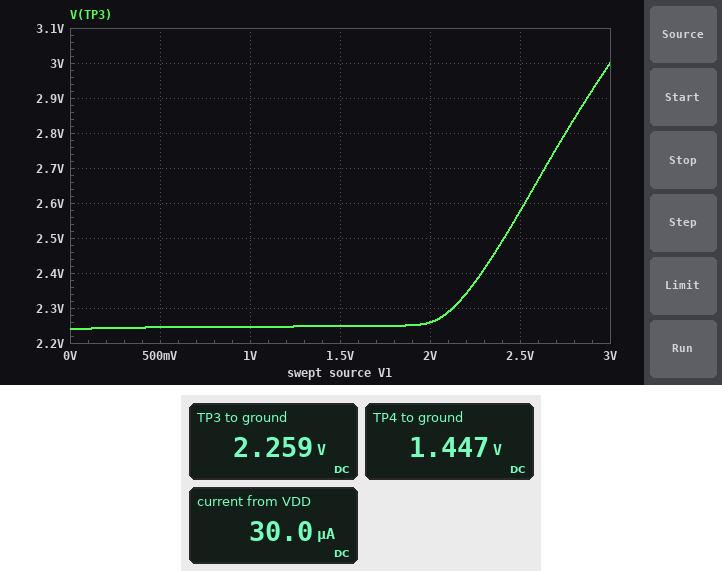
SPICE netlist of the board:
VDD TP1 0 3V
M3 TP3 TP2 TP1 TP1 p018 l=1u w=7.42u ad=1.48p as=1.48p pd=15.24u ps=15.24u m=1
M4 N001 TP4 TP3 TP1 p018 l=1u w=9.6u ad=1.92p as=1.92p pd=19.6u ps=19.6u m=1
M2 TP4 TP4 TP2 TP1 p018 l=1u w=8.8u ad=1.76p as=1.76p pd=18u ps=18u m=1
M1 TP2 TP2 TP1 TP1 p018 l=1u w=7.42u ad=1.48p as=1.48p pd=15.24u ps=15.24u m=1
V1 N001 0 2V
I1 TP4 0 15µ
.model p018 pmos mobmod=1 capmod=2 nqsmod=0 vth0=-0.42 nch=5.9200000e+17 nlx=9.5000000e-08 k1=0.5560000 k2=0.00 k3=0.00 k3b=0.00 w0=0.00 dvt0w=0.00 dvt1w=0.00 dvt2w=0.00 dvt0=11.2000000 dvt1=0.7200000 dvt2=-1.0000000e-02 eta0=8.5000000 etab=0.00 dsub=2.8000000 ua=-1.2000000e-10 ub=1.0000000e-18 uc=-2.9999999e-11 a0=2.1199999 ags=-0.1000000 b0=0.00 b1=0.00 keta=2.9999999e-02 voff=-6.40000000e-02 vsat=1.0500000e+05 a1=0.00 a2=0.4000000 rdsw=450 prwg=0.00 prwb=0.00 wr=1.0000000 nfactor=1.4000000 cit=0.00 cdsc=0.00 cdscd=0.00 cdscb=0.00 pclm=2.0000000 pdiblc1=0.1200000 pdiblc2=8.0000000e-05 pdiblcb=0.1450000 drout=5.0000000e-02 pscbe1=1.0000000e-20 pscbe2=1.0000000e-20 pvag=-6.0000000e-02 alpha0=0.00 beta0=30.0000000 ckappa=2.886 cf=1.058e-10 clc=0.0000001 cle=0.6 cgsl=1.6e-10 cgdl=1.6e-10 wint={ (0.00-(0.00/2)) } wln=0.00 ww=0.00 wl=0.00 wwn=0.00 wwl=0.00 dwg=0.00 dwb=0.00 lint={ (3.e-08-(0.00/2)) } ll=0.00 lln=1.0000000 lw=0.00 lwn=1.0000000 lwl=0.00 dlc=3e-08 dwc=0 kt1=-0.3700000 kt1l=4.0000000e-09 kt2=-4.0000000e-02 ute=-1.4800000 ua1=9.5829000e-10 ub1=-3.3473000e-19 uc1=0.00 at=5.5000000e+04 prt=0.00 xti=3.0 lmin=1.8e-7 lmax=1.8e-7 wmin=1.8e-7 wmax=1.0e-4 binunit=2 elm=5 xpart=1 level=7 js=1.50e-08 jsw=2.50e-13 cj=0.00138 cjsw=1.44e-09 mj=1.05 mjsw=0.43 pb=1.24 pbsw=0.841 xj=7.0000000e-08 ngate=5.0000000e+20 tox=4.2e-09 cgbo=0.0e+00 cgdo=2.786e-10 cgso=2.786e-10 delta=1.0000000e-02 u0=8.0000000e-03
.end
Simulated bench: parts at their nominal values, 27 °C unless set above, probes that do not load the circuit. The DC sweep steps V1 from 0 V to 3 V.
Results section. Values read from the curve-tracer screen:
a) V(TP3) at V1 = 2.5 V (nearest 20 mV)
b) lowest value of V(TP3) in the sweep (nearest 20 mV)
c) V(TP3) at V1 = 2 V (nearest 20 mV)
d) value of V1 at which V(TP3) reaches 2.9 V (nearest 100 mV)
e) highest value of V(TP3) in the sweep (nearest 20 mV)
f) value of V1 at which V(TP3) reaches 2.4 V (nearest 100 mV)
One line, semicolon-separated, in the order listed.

2.58 V; 2.24 V; 2.26 V; 2.9 V; 3.00 V; 2.3 V
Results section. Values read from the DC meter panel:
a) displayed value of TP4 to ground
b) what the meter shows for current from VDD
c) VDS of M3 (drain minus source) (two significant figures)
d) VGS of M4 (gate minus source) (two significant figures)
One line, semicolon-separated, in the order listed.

1.447 V; 30.0 µA; -740 mV; -810 mV
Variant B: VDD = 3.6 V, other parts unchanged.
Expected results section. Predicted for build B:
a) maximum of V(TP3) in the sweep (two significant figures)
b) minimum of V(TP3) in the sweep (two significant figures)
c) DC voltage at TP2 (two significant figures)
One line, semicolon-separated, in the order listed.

3.1 V; 2.8 V; 2.9 V
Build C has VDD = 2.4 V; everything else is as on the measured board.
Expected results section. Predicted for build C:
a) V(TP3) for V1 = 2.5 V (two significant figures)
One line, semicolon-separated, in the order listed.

2.5 V
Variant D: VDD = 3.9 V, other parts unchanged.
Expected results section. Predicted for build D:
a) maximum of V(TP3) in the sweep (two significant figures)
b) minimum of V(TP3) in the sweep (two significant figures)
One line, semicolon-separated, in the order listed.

3.2 V; 3.1 V
